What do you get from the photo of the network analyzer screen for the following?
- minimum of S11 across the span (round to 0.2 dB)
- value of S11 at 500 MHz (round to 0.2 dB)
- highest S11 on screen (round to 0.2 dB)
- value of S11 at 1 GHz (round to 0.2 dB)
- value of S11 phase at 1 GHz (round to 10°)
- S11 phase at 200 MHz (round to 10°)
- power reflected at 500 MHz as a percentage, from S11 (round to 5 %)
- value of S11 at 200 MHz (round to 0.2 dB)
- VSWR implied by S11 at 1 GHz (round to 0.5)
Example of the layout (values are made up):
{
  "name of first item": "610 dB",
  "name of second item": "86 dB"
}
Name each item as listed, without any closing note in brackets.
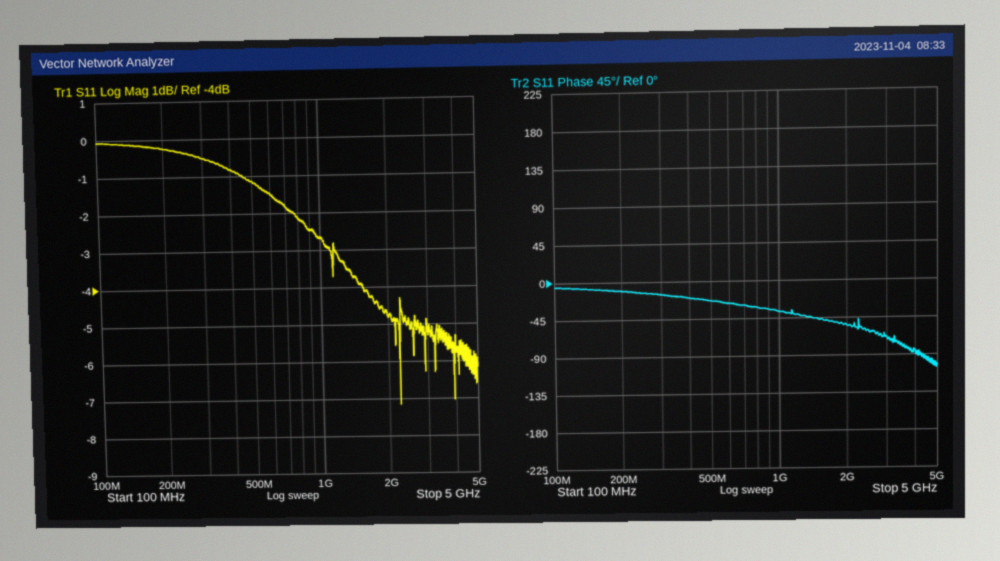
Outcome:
{
  "minimum of S11 across the span": "-7.2 dB",
  "value of S11 at 500 MHz": "-1.2 dB",
  "highest S11 on screen": "0.0 dB",
  "value of S11 at 1 GHz": "-2.6 dB",
  "value of S11 phase at 1 GHz": "-40°",
  "S11 phase at 200 MHz": "-10°",
  "power reflected at 500 MHz as a percentage, from S11": "75 %",
  "value of S11 at 200 MHz": "-0.2 dB",
  "VSWR implied by S11 at 1 GHz": "6.5"
}
